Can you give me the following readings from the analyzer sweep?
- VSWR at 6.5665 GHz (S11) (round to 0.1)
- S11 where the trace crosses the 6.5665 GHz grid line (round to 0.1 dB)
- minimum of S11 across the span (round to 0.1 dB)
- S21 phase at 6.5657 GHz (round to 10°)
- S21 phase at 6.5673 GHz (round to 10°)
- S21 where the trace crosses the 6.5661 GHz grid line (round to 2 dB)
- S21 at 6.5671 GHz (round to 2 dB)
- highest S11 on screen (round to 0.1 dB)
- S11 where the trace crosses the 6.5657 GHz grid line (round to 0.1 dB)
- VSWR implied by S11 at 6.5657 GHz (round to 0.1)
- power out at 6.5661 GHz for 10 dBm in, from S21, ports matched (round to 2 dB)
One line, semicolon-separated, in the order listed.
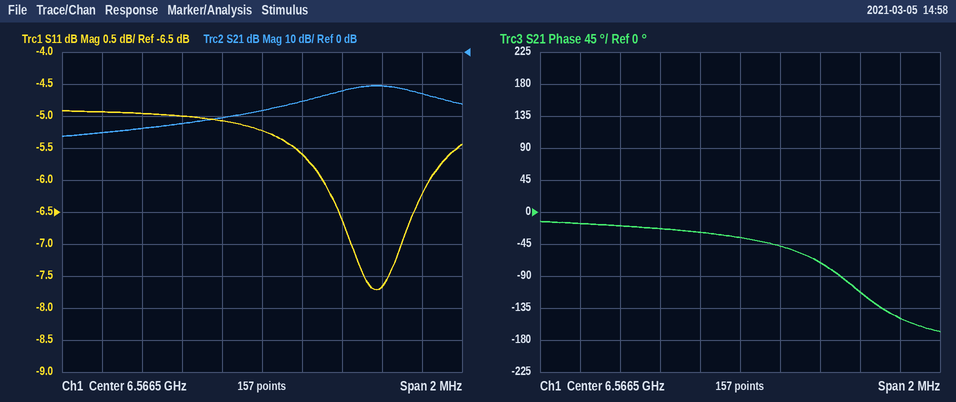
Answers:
3.4; -5.2 dB; -7.7 dB; -20°; -150°; -22 dB; -10 dB; -4.9 dB; -4.9 dB; 3.6; -12 dBm
